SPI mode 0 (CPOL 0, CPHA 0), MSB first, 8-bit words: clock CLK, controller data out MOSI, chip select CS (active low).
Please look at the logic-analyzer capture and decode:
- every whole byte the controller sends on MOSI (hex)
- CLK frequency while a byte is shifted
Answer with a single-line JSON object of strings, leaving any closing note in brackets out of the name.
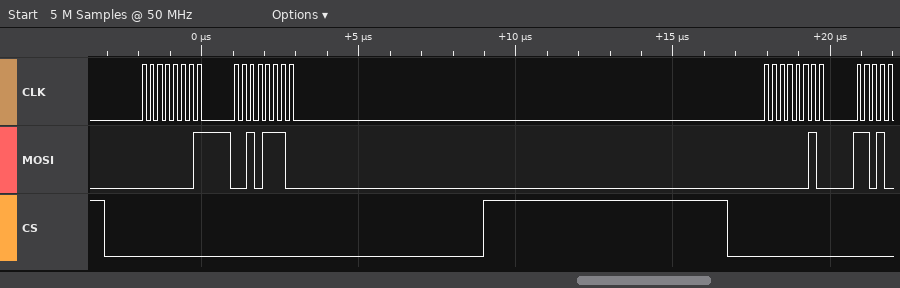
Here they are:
{"every whole byte the controller sends on MOSI": "01 2E 02", "CLK frequency while a byte is shifted": "4 MHz"}
